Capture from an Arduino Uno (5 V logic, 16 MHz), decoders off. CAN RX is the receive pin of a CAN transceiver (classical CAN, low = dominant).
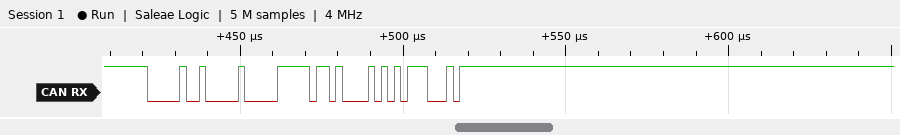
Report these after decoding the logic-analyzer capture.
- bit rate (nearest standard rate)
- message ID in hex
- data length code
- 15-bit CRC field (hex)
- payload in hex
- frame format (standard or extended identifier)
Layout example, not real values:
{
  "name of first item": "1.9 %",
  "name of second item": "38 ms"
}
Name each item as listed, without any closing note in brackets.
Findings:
{
  "bit rate": "500 kbit/s",
  "message ID in hex": "0x010",
  "data length code": "1",
  "15-bit CRC field": "0x0AB8",
  "payload in hex": "FA",
  "frame format": "standard"
}
